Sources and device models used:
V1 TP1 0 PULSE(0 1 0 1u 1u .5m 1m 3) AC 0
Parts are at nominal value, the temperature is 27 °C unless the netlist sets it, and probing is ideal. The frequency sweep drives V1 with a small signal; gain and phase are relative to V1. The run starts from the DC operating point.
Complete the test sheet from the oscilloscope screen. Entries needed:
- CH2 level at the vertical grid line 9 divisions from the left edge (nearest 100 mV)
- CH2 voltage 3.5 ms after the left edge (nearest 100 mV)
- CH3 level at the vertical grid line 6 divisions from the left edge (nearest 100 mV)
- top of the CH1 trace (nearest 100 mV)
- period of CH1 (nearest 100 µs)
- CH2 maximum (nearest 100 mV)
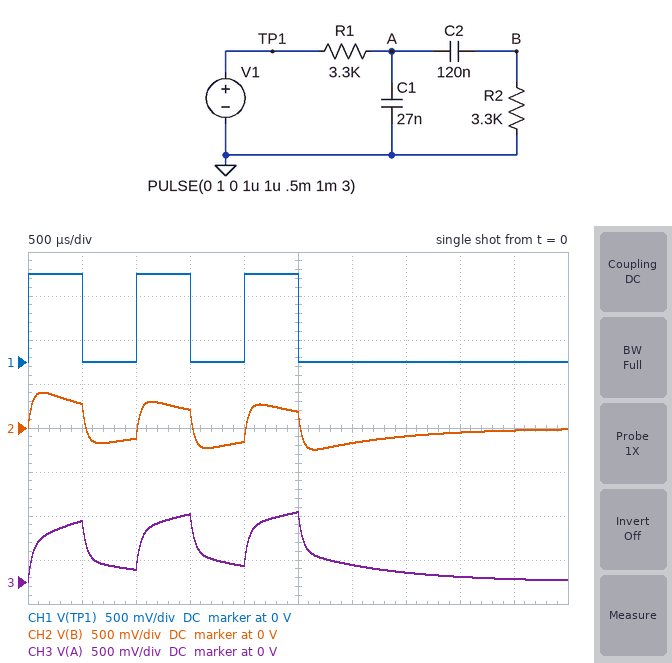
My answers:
0 V
-100 mV
200 mV
1.0 V
1.0 ms
400 mV
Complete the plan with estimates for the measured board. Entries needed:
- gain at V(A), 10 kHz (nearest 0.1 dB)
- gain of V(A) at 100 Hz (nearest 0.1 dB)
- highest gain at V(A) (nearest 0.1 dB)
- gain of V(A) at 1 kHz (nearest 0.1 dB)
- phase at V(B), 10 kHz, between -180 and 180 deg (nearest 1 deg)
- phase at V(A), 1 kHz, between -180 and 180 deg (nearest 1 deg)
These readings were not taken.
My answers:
-15.5 dB
-0.8 dB
0 dB
-6.3 dB
-68 deg
-26 deg
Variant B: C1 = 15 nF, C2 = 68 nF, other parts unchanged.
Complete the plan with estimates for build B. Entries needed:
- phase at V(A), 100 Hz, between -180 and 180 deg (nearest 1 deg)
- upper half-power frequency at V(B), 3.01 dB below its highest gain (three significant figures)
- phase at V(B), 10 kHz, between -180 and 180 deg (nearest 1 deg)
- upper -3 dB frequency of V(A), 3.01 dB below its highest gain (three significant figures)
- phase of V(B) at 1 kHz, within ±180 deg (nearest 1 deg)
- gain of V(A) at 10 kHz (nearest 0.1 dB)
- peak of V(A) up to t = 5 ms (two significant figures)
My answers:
-9 deg
7.45 kHz
-54 deg
448 Hz
10 deg
-11.5 dB
860 mV
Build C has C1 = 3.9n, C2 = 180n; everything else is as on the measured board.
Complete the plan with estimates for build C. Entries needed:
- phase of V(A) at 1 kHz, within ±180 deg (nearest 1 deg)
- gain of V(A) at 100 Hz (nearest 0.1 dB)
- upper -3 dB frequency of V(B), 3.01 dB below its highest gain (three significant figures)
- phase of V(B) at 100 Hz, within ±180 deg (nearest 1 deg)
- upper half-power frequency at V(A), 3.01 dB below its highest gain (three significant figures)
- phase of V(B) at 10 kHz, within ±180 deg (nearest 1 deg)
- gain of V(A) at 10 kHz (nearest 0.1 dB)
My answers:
-10 deg
-1.4 dB
25.1 kHz
53 deg
187 Hz
-21 deg
-6.7 dB
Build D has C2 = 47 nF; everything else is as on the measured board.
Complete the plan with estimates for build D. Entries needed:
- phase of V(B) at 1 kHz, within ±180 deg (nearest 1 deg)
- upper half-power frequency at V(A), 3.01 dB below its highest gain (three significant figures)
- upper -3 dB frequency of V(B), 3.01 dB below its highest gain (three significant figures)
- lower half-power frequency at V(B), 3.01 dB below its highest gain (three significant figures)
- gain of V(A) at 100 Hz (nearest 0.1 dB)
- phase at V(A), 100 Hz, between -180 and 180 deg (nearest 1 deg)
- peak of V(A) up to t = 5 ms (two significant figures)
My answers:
10 deg
543 Hz
4.97 kHz
369 Hz
-0.2 dB
-9 deg
870 mV
